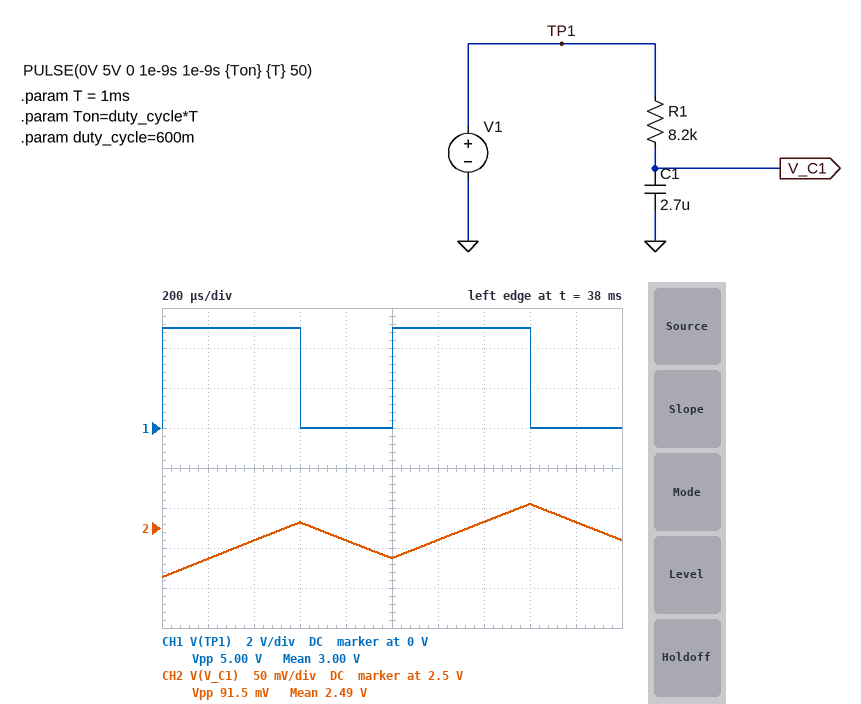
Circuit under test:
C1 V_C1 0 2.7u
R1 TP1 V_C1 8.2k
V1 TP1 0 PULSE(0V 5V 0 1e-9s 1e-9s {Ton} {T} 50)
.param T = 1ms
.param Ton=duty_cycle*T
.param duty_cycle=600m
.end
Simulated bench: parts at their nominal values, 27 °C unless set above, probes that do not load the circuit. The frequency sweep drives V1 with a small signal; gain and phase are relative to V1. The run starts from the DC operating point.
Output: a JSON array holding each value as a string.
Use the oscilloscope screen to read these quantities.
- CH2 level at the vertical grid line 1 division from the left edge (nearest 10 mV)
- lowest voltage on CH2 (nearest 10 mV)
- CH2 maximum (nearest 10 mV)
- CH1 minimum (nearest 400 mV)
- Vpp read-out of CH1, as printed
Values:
["2.46 V", "2.44 V", "2.53 V", "0 V", "5.00 V"]
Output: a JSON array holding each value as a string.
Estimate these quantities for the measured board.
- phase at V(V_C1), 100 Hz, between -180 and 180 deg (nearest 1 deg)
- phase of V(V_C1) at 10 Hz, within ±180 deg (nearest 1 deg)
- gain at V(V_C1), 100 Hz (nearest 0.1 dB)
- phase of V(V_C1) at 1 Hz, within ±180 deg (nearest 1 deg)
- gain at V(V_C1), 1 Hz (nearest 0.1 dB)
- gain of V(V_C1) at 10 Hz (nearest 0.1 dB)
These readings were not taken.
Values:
["-86 deg", "-54 deg", "-22.9 dB", "-8 deg", "-0.1 dB", "-4.7 dB"]
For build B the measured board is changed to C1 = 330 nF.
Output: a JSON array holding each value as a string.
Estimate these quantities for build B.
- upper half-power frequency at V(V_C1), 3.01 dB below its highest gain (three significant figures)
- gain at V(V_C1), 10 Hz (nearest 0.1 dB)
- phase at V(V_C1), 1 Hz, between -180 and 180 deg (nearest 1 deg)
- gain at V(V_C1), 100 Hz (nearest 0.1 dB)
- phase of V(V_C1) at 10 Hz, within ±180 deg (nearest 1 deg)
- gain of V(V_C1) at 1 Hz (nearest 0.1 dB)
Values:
["58.8 Hz", "-0.1 dB", "-1 deg", "-5.9 dB", "-10 deg", "0 dB"]
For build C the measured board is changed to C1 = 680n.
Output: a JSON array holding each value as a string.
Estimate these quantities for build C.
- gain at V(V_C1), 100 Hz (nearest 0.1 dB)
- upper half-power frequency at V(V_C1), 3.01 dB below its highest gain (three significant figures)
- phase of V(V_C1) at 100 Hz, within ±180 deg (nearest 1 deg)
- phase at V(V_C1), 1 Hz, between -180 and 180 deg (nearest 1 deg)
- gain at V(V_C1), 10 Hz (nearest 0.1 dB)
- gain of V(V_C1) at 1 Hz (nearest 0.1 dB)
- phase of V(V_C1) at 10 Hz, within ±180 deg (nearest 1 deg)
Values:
["-11.2 dB", "28.5 Hz", "-74 deg", "-2 deg", "-0.5 dB", "0 dB", "-19 deg"]
